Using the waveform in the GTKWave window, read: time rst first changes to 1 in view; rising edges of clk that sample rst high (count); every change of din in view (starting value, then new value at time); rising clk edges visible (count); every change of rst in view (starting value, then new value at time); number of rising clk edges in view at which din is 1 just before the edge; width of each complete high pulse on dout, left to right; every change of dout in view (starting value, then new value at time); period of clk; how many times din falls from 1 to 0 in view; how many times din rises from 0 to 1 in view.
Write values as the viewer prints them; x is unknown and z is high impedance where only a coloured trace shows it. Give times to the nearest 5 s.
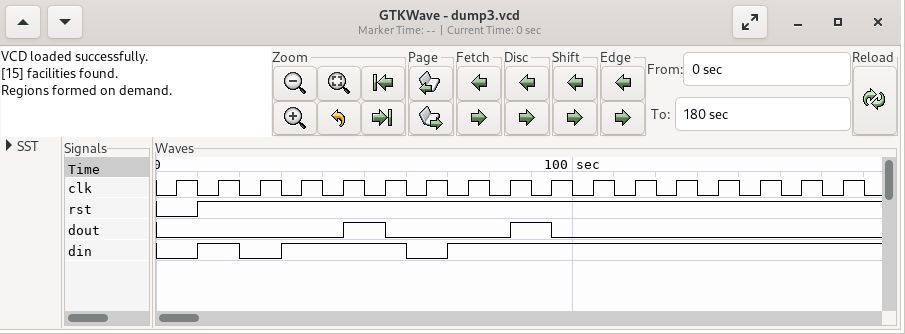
10 s
16
0, 1 at 10 s, 0 at 20 s, 1 at 30 s, 0 at 60 s, 1 at 70 s
17
0, 1 at 10 s
14
10 s, 10 s
0, 1 at 45 s, 0 at 55 s, 1 at 85 s, 0 at 95 s
10 s
2
3
